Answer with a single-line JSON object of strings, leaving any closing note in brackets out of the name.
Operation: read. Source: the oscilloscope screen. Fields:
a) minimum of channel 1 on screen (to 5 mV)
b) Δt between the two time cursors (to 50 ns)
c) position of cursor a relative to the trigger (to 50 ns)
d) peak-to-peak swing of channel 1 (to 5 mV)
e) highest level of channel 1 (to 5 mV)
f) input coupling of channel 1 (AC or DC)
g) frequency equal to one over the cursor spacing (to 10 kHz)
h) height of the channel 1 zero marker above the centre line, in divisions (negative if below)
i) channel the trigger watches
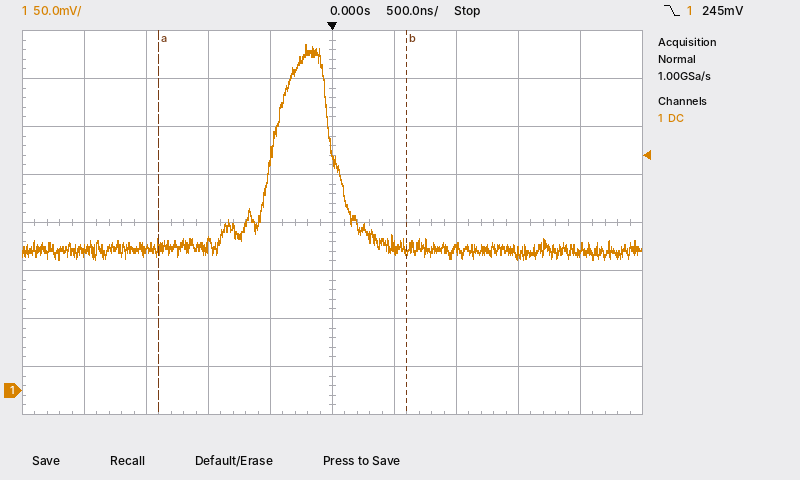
{"minimum of channel 1 on screen": "135 mV", "Δt between the two time cursors": "2.00 µs", "position of cursor a relative to the trigger": "-1.40 µs", "peak-to-peak swing of channel 1": "225 mV", "highest level of channel 1": "360 mV", "input coupling of channel 1": "DC", "frequency equal to one over the cursor spacing": "500 kHz", "height of the channel 1 zero marker above the centre line, in divisions": "-3.5 div", "channel the trigger watches": "channel 1"}
